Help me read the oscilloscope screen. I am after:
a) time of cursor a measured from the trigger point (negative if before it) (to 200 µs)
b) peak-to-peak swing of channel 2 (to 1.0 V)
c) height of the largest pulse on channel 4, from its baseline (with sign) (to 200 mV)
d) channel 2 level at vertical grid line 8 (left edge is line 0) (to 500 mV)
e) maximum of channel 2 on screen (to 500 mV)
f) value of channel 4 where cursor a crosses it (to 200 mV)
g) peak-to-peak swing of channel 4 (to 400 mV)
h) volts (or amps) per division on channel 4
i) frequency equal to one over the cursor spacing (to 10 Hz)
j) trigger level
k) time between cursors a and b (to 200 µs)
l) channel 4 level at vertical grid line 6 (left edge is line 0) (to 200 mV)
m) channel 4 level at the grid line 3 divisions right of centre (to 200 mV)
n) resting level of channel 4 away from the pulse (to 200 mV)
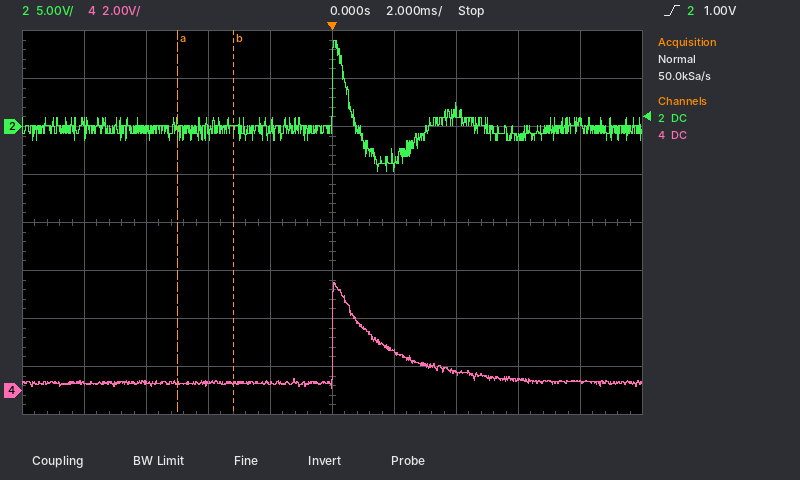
-5.0 ms
14.0 V
+4.2 V
-1.0 V
9.0 V
400 mV
4.4 V
2 V
560 Hz
1.00 V
1.8 ms
1.6 V
400 mV
400 mV
